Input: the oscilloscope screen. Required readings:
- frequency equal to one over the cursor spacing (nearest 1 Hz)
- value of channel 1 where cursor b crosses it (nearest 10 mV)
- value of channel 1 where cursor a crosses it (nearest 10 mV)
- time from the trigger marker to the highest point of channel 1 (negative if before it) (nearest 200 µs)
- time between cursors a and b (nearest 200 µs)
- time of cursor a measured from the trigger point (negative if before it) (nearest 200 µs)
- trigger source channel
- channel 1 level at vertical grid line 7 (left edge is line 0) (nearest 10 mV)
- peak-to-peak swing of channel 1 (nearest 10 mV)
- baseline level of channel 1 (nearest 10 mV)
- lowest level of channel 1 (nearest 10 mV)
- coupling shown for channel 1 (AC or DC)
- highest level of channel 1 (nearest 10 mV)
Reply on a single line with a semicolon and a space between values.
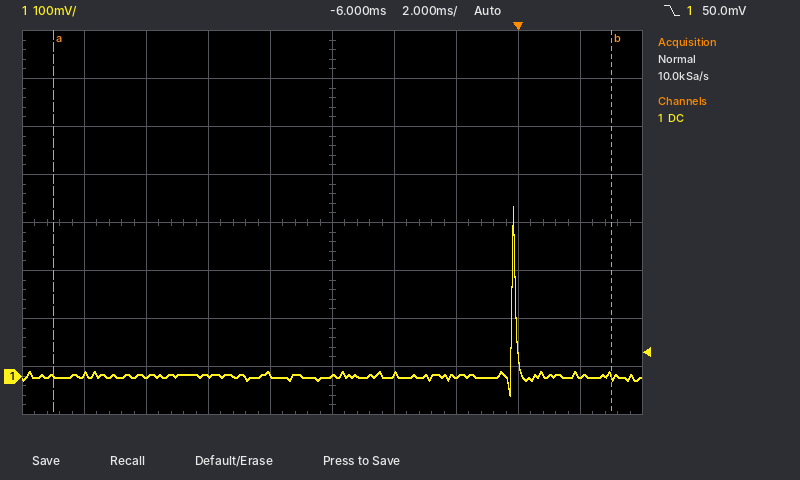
56 Hz; 0 mV; 0 mV; -200 µs; 18.0 ms; -15.0 ms; channel 1; 0 mV; 390 mV; 0 mV; -40 mV; DC; 350 mV
